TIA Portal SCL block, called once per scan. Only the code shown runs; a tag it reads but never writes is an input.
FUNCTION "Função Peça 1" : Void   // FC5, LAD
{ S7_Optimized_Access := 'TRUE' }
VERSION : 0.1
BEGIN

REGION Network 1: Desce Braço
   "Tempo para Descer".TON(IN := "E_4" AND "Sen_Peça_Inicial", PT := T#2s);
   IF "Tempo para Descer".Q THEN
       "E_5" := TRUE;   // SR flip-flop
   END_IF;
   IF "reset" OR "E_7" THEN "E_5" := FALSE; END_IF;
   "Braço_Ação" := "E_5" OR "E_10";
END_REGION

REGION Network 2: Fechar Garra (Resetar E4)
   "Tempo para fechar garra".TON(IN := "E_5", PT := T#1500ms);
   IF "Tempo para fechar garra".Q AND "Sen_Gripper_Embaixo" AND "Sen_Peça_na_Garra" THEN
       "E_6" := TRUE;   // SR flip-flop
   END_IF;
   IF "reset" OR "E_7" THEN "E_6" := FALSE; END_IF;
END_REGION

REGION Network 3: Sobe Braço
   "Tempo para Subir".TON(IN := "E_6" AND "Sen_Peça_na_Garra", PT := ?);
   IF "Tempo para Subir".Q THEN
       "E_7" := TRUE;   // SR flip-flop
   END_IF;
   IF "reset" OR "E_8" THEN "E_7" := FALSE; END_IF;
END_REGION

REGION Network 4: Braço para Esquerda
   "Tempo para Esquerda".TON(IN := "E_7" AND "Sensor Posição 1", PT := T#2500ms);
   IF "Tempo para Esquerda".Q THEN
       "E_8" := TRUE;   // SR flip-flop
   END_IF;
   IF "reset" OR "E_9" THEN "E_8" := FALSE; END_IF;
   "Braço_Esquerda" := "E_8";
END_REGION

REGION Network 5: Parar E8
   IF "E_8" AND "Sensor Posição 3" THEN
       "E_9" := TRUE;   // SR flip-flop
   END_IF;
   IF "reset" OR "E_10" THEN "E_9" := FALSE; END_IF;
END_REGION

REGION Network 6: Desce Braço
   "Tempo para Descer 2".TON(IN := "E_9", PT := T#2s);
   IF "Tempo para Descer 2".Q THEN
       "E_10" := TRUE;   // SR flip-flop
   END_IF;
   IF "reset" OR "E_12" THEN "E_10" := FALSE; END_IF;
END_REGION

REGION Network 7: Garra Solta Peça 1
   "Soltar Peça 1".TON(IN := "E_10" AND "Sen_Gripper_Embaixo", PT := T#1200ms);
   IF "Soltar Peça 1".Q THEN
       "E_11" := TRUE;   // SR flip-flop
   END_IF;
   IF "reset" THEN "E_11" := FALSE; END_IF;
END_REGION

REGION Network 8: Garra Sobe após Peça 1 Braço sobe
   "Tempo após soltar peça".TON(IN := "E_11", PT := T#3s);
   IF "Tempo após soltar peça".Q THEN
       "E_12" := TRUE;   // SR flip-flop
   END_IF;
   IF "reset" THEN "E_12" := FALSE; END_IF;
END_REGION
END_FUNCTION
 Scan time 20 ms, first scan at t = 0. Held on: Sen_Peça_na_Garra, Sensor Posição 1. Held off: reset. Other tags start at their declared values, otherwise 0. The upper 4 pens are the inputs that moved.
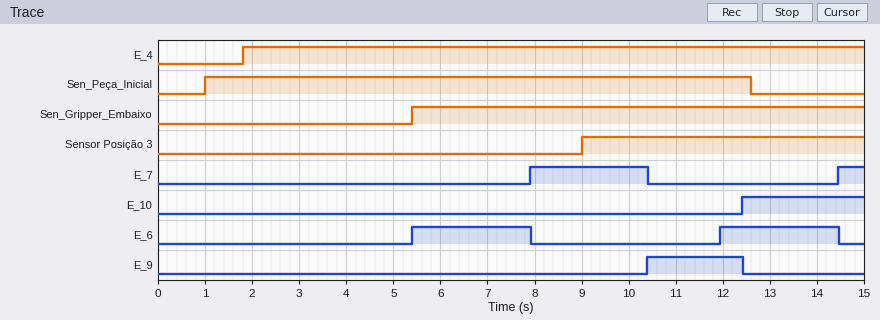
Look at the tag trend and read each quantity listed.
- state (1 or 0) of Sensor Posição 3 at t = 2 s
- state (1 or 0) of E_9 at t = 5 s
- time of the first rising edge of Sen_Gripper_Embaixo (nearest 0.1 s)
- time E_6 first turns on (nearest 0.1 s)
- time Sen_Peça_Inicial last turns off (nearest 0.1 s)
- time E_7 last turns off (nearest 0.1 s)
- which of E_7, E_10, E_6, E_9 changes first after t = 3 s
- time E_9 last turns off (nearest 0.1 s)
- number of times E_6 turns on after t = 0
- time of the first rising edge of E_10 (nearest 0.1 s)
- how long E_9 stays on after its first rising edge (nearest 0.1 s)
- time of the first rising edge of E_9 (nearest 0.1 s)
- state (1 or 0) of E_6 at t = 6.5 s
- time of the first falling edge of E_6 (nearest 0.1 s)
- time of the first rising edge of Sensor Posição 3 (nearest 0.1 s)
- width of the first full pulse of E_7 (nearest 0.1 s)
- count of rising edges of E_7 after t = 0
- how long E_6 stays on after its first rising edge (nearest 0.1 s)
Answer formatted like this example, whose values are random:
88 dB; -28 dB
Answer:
0; 0; 5.4 s; 5.4 s; 12.6 s; 10.4 s; E_6; 12.4 s; 2; 12.4 s; 2.0 s; 10.4 s; 1; 7.9 s; 9.0 s; 2.5 s; 2; 2.5 s
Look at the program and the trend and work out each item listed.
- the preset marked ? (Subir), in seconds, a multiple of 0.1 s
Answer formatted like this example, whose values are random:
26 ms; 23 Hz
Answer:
2.5 s
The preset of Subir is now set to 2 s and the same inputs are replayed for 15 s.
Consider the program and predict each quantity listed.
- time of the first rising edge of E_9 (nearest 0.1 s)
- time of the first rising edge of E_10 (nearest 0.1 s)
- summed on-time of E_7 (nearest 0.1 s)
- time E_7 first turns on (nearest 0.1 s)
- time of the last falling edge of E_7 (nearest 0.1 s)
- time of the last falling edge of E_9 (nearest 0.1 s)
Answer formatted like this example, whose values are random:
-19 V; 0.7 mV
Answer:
9.9 s; 11.9 s; 4.1 s; 7.4 s; 9.9 s; 11.9 s
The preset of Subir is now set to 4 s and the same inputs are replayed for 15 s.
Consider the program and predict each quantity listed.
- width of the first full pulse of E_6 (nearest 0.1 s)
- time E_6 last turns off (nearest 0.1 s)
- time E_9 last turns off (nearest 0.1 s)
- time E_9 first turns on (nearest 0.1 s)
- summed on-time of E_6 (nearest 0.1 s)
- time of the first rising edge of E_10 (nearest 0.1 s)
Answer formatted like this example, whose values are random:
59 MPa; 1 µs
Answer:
4.0 s; 9.4 s; 13.9 s; 11.9 s; 5.6 s; 13.9 s
